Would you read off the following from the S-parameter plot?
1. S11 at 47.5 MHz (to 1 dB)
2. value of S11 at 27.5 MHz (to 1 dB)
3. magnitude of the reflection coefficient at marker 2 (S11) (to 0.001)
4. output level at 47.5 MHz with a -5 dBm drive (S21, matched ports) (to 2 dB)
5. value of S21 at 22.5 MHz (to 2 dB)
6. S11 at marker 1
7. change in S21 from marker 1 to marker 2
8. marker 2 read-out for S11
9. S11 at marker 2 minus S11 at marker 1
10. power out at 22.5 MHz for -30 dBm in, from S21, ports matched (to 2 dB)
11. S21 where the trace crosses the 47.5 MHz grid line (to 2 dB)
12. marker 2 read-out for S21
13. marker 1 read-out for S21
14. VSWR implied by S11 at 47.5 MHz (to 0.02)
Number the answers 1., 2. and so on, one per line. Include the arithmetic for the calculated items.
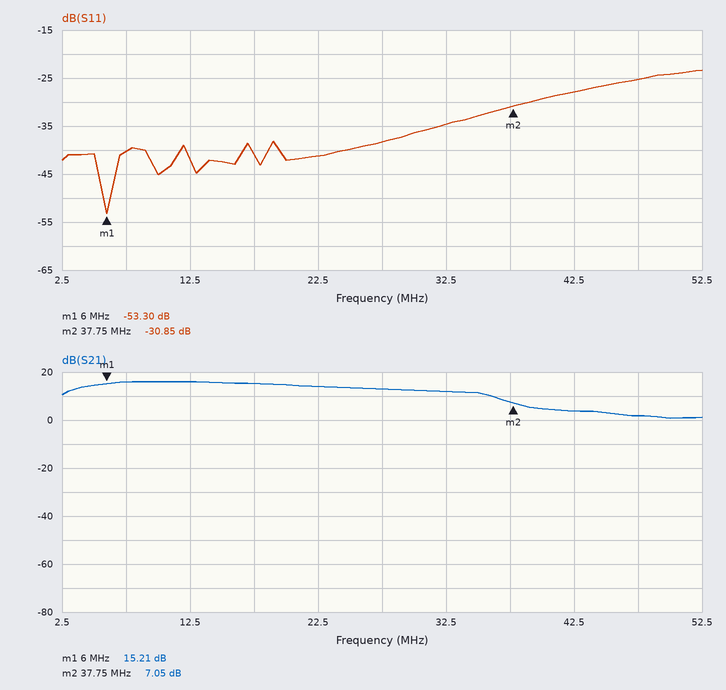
1. -25 dB
2. -38 dB
3. 10^(-30.85/20) ≈ 0.029
4. -5 dBm + (2 dB) = -4 dBm
5. 14 dB
6. -53.30 dB
7. 7.05 − (15.21) = -8.16 dB
8. -30.85 dB
9. -30.85 − (-53.3) = 22.45 dB
10. -30 dBm + (14 dB) = -16 dBm
11. 2 dB
12. 7.05 dB
13. 15.21 dB
14. |Γ| = 10^(-25/20) = 0.0562; VSWR = (1 + 0.0562)/(1 − 0.0562) ≈ 1.12
